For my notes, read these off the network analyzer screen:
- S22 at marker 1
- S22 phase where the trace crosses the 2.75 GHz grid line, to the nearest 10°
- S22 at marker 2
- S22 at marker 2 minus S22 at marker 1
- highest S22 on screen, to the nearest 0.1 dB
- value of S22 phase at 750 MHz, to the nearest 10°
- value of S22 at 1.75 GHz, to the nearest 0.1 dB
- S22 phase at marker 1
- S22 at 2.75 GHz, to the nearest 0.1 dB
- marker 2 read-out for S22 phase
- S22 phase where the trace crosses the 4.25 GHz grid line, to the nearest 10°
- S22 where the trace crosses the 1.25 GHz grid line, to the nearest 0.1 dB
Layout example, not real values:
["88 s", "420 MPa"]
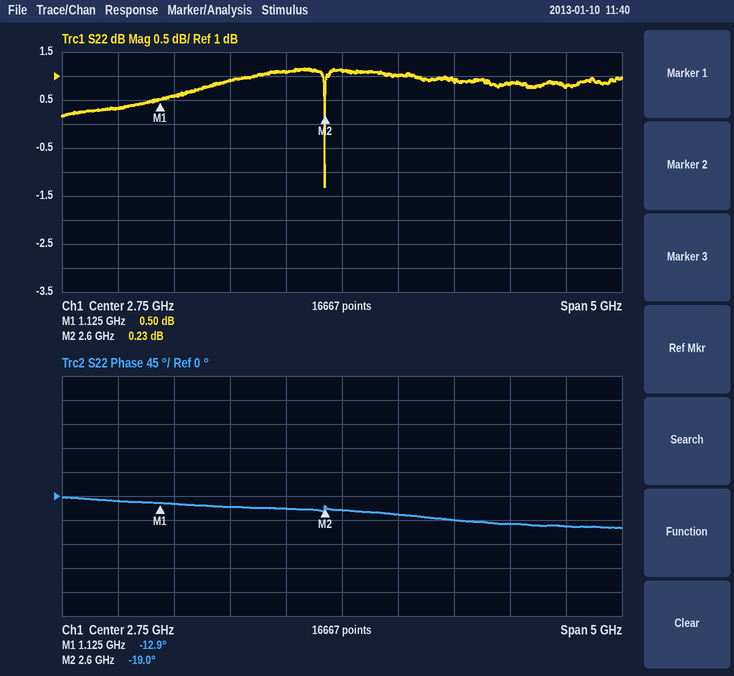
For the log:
["0.50 dB", "-30°", "0.23 dB", "-0.27 dB", "1.2 dB", "-10°", "0.9 dB", "-12.9°", "1.1 dB", "-19.0°", "-50°", "0.6 dB"]
